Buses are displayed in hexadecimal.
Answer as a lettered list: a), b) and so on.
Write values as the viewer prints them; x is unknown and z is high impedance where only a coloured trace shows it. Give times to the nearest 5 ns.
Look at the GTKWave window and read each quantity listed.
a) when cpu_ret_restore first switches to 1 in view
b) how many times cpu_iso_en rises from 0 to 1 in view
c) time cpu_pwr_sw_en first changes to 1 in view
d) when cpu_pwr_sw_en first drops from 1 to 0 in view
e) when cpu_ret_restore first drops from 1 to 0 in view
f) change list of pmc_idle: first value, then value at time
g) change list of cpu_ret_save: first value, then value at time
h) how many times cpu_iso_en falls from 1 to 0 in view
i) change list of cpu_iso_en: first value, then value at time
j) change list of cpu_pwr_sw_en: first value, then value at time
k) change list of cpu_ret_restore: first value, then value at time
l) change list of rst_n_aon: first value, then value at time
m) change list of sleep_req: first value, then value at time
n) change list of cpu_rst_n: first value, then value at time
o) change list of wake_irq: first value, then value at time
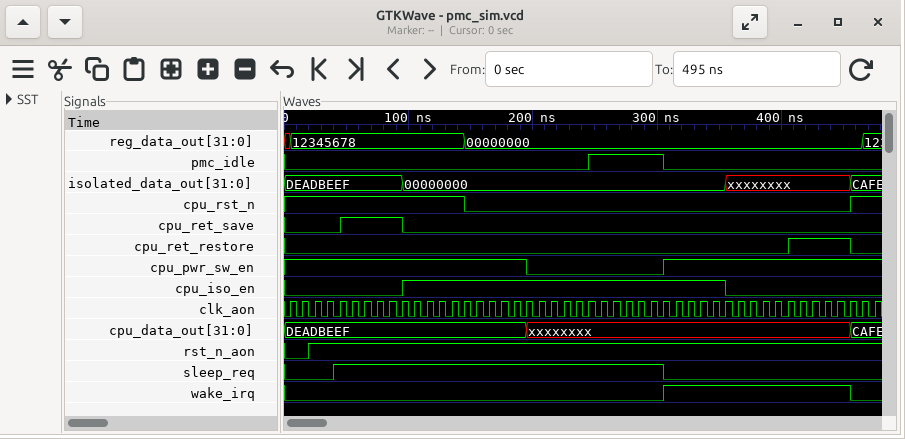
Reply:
a) 405 ns
b) 1
c) 305 ns
d) 195 ns
e) 455 ns
f) 0, 1 at 245 ns, 0 at 305 ns
g) 0, 1 at 45 ns, 0 at 95 ns
h) 1
i) 0, 1 at 95 ns, 0 at 355 ns
j) 1, 0 at 195 ns, 1 at 305 ns
k) 0, 1 at 405 ns, 0 at 455 ns
l) 0, 1 at 20 ns
m) 0, 1 at 40 ns, 0 at 305 ns
n) 1, 0 at 145 ns, 1 at 455 ns
o) 0, 1 at 305 ns, 0 at 455 ns
